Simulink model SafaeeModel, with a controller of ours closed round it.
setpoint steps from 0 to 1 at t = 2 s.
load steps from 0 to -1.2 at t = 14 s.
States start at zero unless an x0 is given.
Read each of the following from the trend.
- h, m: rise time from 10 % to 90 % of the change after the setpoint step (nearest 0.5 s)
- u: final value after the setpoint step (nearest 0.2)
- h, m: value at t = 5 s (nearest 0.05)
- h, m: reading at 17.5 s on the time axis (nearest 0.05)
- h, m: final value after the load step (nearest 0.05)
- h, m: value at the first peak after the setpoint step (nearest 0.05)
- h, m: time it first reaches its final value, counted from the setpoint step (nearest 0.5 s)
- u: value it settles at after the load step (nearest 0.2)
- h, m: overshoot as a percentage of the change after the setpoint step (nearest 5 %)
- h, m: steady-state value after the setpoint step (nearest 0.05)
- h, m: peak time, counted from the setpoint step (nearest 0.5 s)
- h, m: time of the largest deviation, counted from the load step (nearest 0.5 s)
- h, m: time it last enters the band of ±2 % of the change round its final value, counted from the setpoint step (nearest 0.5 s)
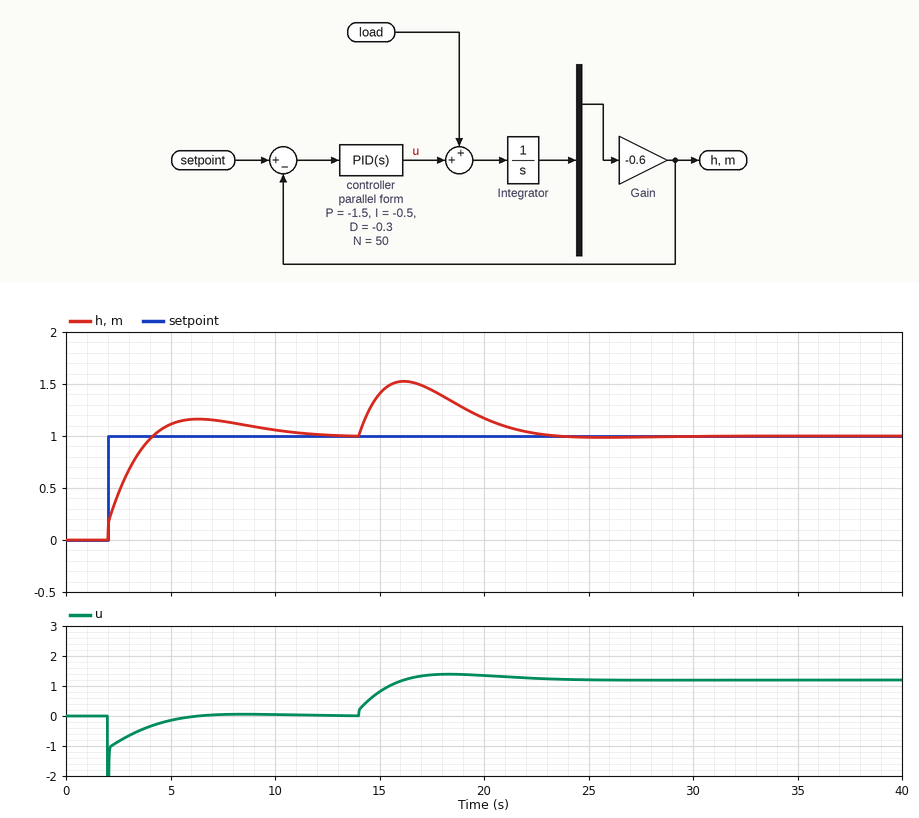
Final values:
1.5 s
0.0
1.10
1.45
1.00
1.15
2.0 s
1.2
15 %
1.00
4.5 s
2.0 s
9.5 s
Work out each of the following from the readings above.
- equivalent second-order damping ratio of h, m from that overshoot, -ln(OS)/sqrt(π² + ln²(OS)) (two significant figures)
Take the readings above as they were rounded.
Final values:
0.52
